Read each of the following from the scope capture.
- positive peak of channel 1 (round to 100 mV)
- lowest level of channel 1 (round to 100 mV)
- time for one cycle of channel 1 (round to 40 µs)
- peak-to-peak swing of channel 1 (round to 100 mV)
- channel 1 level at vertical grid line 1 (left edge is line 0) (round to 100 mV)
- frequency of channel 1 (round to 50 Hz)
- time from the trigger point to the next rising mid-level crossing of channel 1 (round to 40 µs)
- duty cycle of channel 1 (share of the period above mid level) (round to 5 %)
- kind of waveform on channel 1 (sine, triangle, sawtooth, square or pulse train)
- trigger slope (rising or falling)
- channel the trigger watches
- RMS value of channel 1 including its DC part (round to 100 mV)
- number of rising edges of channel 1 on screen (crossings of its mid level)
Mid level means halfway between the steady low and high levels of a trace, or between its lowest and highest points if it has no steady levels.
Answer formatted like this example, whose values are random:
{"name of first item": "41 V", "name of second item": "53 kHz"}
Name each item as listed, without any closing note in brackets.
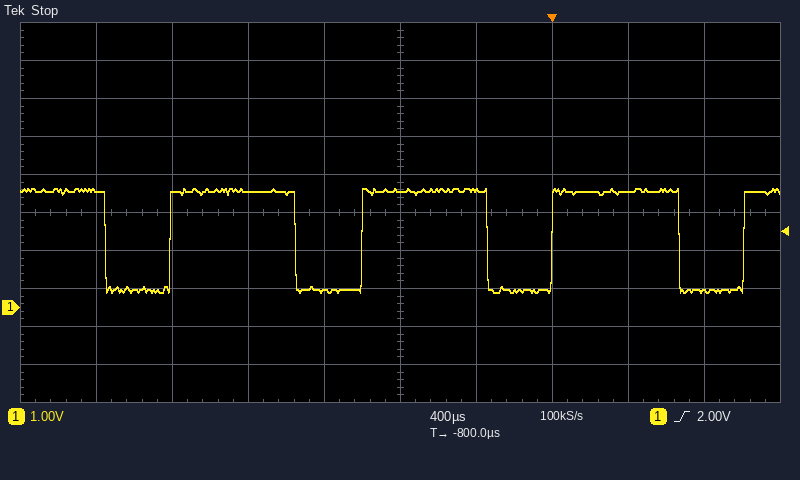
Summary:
{"positive peak of channel 1": "3.1 V", "lowest level of channel 1": "400 mV", "time for one cycle of channel 1": "1.00 ms", "peak-to-peak swing of channel 1": "2.7 V", "channel 1 level at vertical grid line 1 (left edge is line 0)": "3.1 V", "frequency of channel 1": "1.00 kHz", "time from the trigger point to the next rising mid-level crossing of channel 1": "1.00 ms", "duty cycle of channel 1 (share of the period above mid level)": "65 %", "kind of waveform on channel 1": "pulse train", "trigger slope": "rising", "channel the trigger watches": "channel 1", "RMS value of channel 1 including its DC part": "2.5 V", "number of rising edges of channel 1 on screen": "4"}
